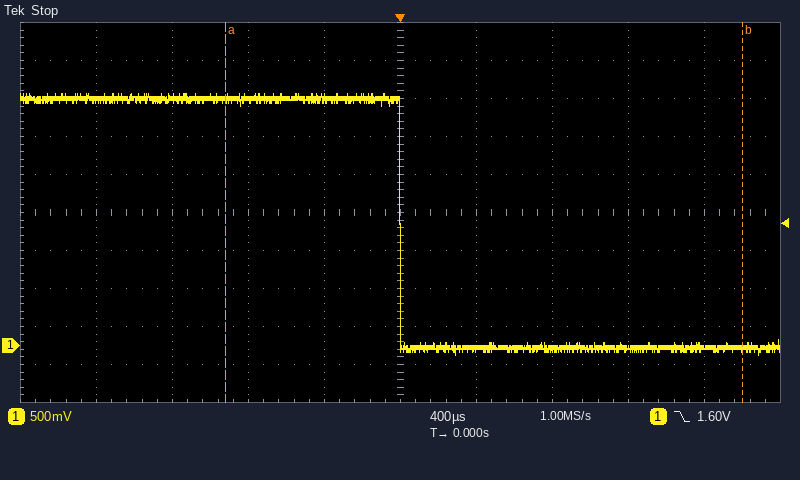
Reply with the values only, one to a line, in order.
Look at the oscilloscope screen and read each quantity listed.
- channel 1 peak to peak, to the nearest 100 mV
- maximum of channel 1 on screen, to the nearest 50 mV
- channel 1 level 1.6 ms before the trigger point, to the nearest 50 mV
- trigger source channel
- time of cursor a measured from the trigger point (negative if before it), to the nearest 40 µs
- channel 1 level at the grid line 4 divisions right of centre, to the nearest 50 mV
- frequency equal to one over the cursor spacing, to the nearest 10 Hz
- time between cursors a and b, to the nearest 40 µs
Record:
3.40 V
3.30 V
3.25 V
channel 1
-920 µs
-50 mV
370 Hz
2.72 ms
